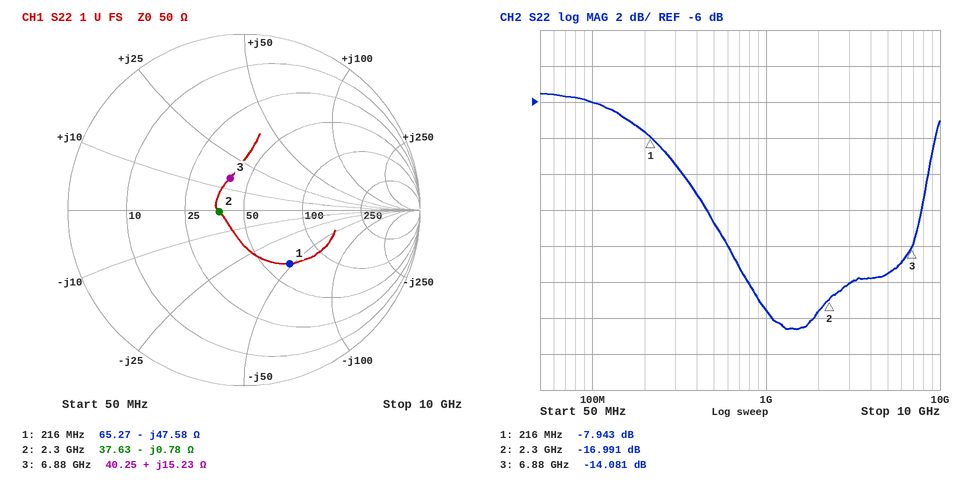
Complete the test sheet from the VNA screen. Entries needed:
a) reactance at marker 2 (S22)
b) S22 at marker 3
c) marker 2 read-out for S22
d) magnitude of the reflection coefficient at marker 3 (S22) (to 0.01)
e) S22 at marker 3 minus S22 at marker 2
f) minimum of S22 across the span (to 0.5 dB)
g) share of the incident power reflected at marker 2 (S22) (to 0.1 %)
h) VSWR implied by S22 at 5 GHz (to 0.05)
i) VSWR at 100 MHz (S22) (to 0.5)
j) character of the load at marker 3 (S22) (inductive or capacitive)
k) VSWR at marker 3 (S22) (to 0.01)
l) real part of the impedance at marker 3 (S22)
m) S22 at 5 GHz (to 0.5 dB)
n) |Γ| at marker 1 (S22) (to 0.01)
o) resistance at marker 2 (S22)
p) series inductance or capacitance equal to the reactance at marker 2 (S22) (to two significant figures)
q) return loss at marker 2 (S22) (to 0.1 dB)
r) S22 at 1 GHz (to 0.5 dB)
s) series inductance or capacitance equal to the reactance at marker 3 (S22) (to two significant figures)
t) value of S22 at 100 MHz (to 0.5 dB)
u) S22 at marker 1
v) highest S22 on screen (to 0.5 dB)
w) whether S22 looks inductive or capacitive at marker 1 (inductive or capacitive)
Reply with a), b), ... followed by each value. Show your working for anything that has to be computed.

a) -0.78 Ω
b) -14.081 dB
c) -16.991 dB
d) 0.20
e) -14.081 − (-16.991) = 2.910 dB
f) -18.5 dB
g) 10^(-16.991/10) ≈ 2.0 %
h) |Γ| = 10^(-15.5/20) = 0.1679; VSWR = (1 + 0.1679)/(1 − 0.1679) ≈ 1.40
i) |Γ| = 10^(-6/20) = 0.5012; VSWR = (1 + 0.5012)/(1 − 0.5012) ≈ 3.0
j) inductive
k) (1 + 0.1977)/(1 − 0.1977) ≈ 1.49
l) 40.25 Ω
m) -15.5 dB
n) 0.40
o) 37.63 Ω
p) C = 1/(2π × 2.3 GHz × 0.78 Ω) ≈ 89 pF
q) 17.0 dB
r) -17.5 dB
s) L = 15.23 Ω/(2π × 6.88 GHz) ≈ 352 pH, so 350 pH to two significant figures
t) -6.0 dB
u) -7.943 dB
v) -5.5 dB
w) capacitive
